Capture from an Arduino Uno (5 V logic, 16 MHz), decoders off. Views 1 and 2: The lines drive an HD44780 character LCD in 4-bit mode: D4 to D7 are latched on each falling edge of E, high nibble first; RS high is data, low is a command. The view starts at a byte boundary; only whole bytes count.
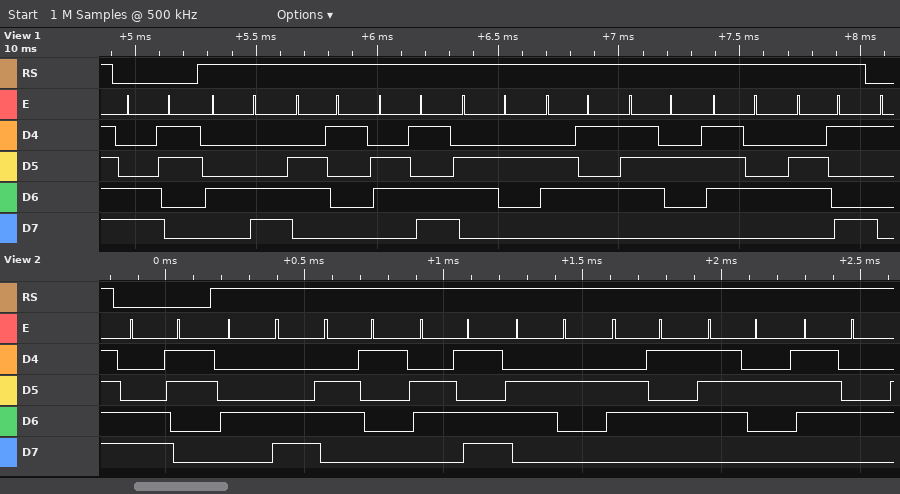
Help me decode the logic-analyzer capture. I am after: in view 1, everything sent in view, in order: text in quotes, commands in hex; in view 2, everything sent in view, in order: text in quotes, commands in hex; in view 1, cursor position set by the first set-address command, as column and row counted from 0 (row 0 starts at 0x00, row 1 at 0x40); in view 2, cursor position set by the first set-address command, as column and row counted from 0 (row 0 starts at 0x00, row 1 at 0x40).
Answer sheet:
0xC3 "Lamberti"
0xC3 "Lambert"
column 3, row 1
column 3, row 1
